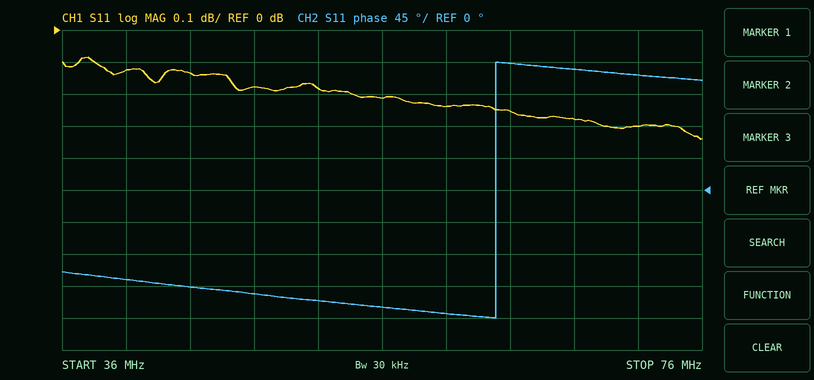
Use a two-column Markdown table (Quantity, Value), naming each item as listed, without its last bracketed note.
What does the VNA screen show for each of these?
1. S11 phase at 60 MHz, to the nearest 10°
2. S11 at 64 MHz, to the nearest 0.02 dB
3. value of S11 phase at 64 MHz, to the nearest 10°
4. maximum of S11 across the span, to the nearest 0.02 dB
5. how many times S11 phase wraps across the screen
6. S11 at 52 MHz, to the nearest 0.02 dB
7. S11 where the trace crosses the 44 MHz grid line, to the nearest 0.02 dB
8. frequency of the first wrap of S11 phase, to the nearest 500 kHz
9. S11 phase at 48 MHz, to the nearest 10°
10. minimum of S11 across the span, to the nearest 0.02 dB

| Quantity | Value |
|---|---|
| S11 phase at 60 MHz, to the nearest 10° | -170° |
| S11 at 64 MHz, to the nearest 0.02 dB | -0.26 dB |
| value of S11 phase at 64 MHz, to the nearest 10° | 180° |
| maximum of S11 across the span, to the nearest 0.02 dB | -0.08 dB |
| how many times S11 phase wraps across the screen | 1 |
| S11 at 52 MHz, to the nearest 0.02 dB | -0.18 dB |
| S11 where the trace crosses the 44 MHz grid line, to the nearest 0.02 dB | -0.14 dB |
| frequency of the first wrap of S11 phase, to the nearest 500 kHz | 63.0 MHz |
| S11 phase at 48 MHz, to the nearest 10° | -150° |
| minimum of S11 across the span, to the nearest 0.02 dB | -0.34 dB |
